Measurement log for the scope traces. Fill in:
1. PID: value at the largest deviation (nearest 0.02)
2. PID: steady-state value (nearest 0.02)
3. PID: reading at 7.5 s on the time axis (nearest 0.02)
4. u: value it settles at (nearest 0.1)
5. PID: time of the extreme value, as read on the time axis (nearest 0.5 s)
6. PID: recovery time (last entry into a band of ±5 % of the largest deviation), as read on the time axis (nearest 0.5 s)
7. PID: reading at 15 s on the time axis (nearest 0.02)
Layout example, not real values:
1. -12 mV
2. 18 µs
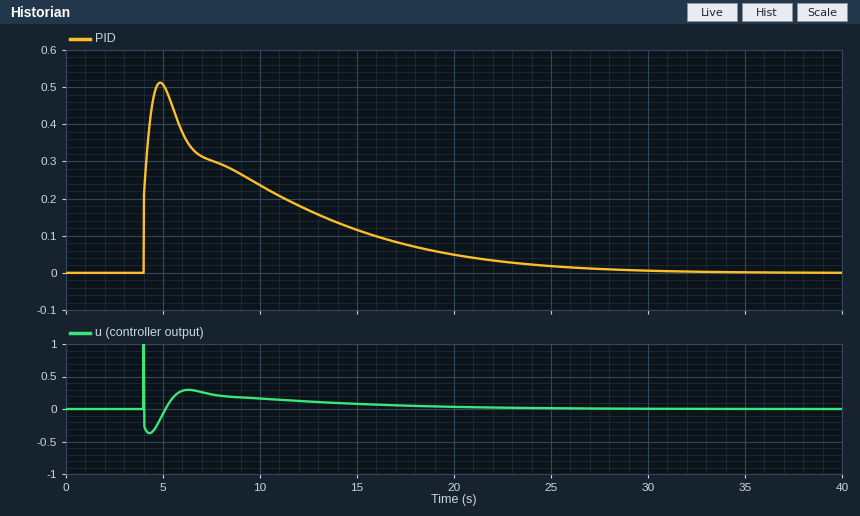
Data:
1. 0.52
2. 0.00
3. 0.30
4. 0.0
5. 5.0 s
6. 23.5 s
7. 0.12
